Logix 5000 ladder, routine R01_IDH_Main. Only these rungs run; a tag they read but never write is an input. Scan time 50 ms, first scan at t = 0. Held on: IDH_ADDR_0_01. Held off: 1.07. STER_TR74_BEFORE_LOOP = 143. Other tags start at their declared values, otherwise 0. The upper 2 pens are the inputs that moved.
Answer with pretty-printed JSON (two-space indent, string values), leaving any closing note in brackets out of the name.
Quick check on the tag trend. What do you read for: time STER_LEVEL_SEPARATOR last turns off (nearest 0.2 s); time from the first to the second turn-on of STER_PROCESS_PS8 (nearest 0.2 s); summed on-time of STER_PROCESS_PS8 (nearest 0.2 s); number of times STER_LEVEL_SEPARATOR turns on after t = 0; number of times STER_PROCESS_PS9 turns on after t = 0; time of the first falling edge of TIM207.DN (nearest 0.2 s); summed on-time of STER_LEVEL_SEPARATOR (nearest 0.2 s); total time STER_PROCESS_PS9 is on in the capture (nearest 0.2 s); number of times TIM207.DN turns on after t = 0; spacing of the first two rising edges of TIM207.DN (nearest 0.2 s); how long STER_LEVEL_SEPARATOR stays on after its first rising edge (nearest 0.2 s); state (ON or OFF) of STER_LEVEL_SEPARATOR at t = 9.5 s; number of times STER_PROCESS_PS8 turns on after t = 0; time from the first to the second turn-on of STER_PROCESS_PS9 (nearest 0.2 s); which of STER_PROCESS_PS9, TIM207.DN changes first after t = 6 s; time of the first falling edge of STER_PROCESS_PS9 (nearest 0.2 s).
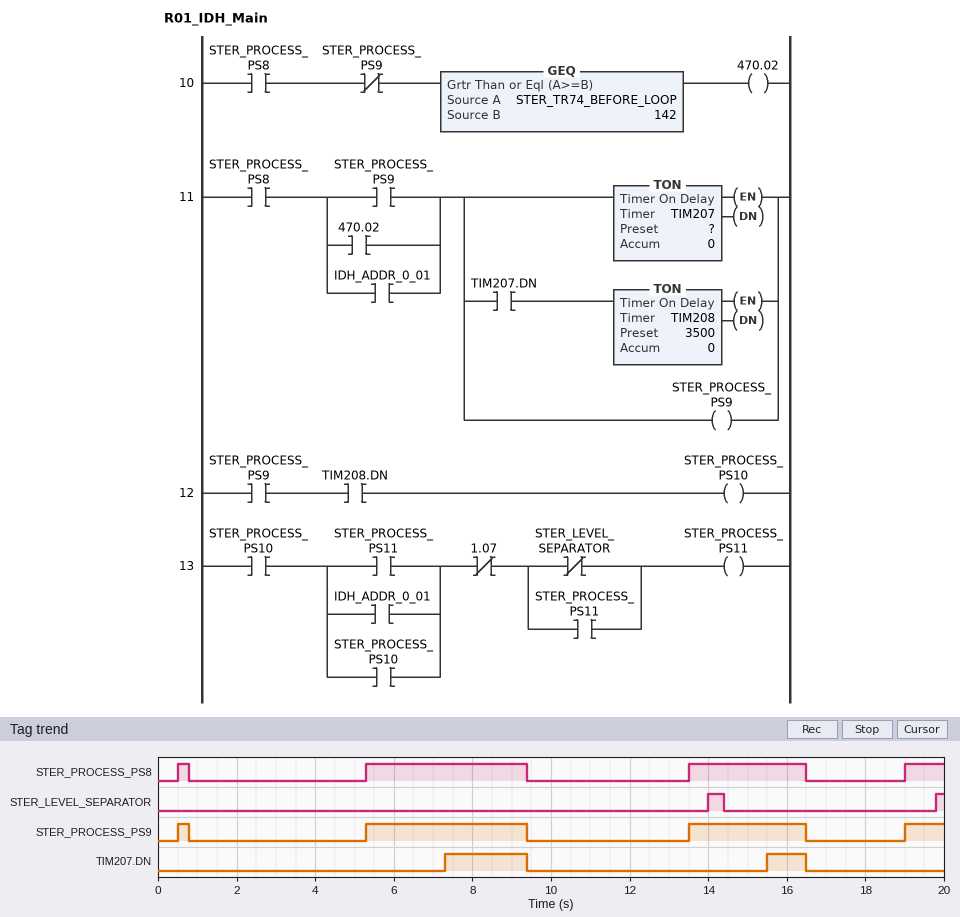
{
  "time STER_LEVEL_SEPARATOR last turns off": "14.4 s",
  "time from the first to the second turn-on of STER_PROCESS_PS8": "4.8 s",
  "summed on-time of STER_PROCESS_PS8": "8.4 s",
  "number of times STER_LEVEL_SEPARATOR turns on after t = 0": "2",
  "number of times STER_PROCESS_PS9 turns on after t = 0": "4",
  "time of the first falling edge of TIM207.DN": "9.4 s",
  "summed on-time of STER_LEVEL_SEPARATOR": "0.6 s",
  "total time STER_PROCESS_PS9 is on in the capture": "8.4 s",
  "number of times TIM207.DN turns on after t = 0": "2",
  "spacing of the first two rising edges of TIM207.DN": "8.2 s",
  "how long STER_LEVEL_SEPARATOR stays on after its first rising edge": "0.4 s",
  "state (ON or OFF) of STER_LEVEL_SEPARATOR at t = 9.5 s": "OFF",
  "number of times STER_PROCESS_PS8 turns on after t = 0": "4",
  "time from the first to the second turn-on of STER_PROCESS_PS9": "4.8 s",
  "which of STER_PROCESS_PS9, TIM207.DN changes first after t = 6 s": "TIM207.DN",
  "time of the first falling edge of STER_PROCESS_PS9": "0.8 s"
}
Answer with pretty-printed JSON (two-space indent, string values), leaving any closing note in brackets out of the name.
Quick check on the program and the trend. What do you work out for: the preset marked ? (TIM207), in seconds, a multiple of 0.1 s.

{
  "the preset marked ? (TIM207), in seconds, a multiple of 0.1 s": "2.0 s"
}
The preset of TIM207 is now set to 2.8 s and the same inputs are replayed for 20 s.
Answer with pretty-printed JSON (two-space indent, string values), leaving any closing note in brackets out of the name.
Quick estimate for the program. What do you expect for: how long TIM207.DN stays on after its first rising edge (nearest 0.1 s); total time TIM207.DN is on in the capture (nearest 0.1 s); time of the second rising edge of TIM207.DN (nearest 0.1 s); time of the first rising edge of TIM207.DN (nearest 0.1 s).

{
  "how long TIM207.DN stays on after its first rising edge": "1.3 s",
  "total time TIM207.DN is on in the capture": "1.5 s",
  "time of the second rising edge of TIM207.DN": "16.3 s",
  "time of the first rising edge of TIM207.DN": "8.1 s"
}
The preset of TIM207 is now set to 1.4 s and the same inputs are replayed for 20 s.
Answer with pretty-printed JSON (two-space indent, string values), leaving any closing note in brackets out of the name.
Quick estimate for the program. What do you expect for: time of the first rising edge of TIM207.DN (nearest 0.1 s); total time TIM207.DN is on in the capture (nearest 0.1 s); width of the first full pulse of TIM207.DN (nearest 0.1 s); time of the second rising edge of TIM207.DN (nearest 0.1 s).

{
  "time of the first rising edge of TIM207.DN": "6.7 s",
  "total time TIM207.DN is on in the capture": "4.3 s",
  "width of the first full pulse of TIM207.DN": "2.7 s",
  "time of the second rising edge of TIM207.DN": "14.9 s"
}
